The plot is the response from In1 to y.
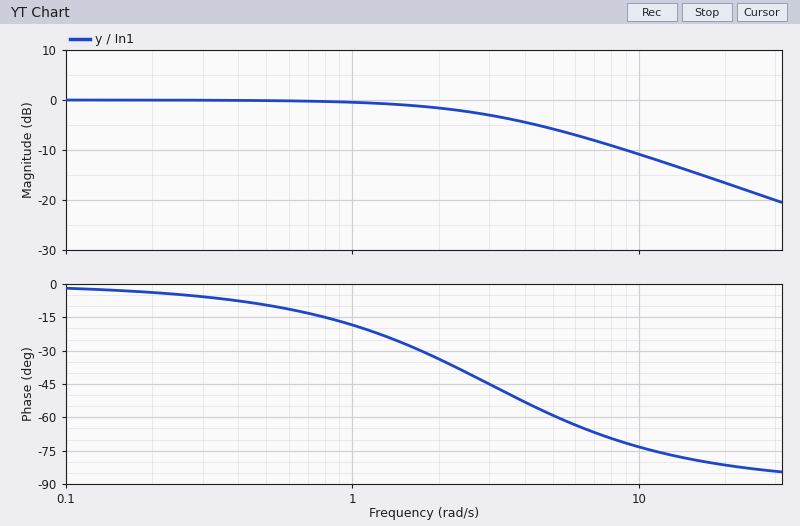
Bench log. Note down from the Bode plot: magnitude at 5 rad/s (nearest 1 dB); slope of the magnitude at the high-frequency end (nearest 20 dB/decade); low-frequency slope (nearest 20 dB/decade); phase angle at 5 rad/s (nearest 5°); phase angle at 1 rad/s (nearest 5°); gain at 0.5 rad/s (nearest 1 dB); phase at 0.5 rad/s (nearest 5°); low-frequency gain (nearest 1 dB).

-6 dB
-20 dB/decade
0 dB/decade
-60°
-20°
0 dB
-10°
0 dB
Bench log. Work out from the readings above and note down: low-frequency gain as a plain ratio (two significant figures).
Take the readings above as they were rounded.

1.0
